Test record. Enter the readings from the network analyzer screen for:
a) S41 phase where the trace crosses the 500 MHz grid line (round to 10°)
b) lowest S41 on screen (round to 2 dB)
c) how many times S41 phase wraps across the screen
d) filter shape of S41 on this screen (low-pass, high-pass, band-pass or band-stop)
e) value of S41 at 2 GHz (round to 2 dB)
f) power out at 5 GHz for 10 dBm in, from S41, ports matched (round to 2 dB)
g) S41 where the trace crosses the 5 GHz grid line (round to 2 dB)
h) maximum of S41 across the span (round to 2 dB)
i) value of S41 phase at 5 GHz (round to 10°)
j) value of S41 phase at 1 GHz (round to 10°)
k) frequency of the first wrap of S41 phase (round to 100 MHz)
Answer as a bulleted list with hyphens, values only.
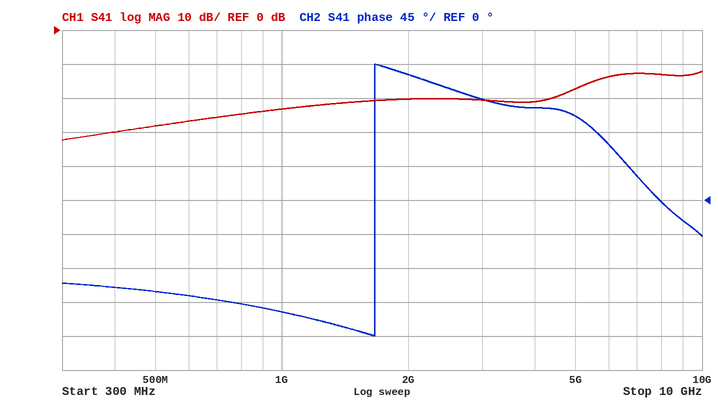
- -120°
- -32 dB
- 1
- high-pass
- -20 dB
- -8 dBm
- -18 dB
- -12 dB
- 110°
- -150°
- 1.7 GHz
